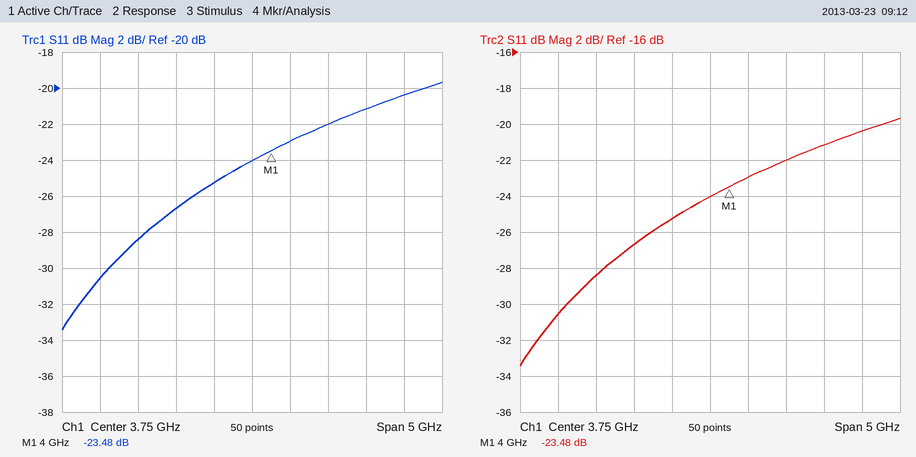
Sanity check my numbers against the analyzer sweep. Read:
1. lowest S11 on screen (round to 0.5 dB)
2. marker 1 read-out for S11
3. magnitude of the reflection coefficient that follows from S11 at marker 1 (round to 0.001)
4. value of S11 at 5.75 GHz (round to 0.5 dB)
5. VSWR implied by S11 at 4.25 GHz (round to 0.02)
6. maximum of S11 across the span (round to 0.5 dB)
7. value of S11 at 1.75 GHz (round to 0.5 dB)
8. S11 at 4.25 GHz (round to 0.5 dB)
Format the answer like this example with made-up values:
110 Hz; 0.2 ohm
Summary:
-33.5 dB; -23.48 dB; 0.067; -20.5 dB; 1.16; -19.5 dB; -30.5 dB; -23.0 dB
